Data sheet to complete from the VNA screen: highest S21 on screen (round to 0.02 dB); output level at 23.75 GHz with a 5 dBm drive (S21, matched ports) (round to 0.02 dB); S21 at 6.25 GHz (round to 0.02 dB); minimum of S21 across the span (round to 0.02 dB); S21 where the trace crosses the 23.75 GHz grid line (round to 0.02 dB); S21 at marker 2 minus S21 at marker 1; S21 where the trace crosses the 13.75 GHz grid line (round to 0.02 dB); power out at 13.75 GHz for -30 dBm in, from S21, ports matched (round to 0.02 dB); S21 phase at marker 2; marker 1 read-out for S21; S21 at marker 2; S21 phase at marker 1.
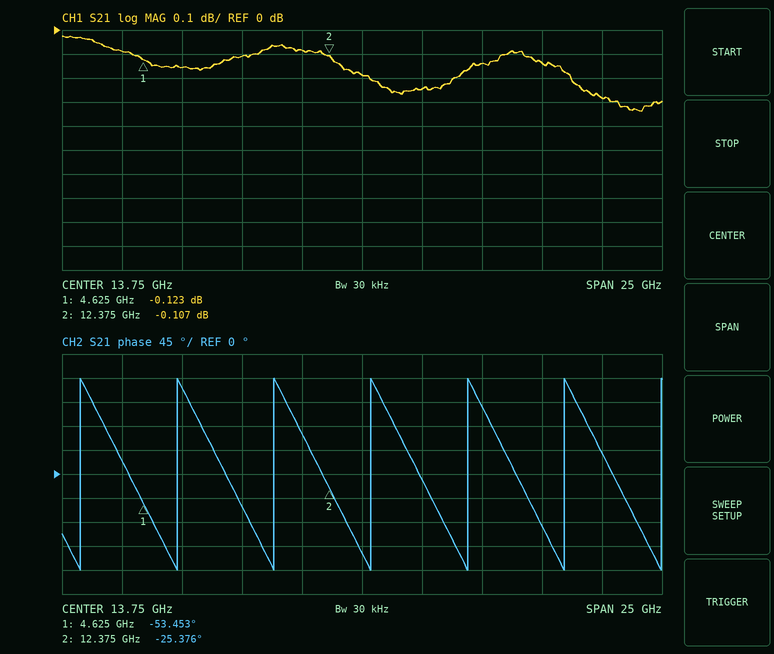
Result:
-0.02 dB
4.72 dBm
-0.16 dB
-0.34 dB
-0.28 dB
0.016 dB
-0.18 dB
-30.18 dBm
-25.376°
-0.123 dB
-0.107 dB
-53.453°
